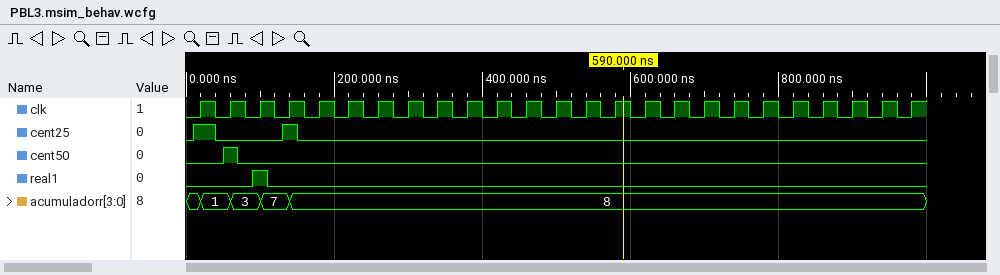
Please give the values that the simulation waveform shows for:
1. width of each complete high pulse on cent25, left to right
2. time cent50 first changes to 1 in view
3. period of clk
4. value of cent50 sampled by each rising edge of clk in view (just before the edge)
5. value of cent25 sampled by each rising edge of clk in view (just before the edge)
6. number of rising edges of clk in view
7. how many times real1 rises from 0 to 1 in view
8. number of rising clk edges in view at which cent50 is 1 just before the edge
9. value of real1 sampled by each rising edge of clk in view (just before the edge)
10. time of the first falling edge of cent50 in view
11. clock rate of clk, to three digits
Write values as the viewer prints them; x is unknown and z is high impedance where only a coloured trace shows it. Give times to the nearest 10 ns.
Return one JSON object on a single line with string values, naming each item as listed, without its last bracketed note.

{"width of each complete high pulse on cent25, left to right": "30 ns, 20 ns", "time cent50 first changes to 1 in view": "50 ns", "period of clk": "40 ns", "value of cent50 sampled by each rising edge of clk in view": "0 1 0 0 0 0 0 0 0 0 0 0 0 0 0 0 0 0 0 0 0 0 0 0 0", "value of cent25 sampled by each rising edge of clk in view": "1 0 0 1 0 0 0 0 0 0 0 0 0 0 0 0 0 0 0 0 0 0 0 0 0", "number of rising edges of clk in view": "25", "how many times real1 rises from 0 to 1 in view": "1", "number of rising clk edges in view at which cent50 is 1 just before the edge": "1", "value of real1 sampled by each rising edge of clk in view": "0 0 1 0 0 0 0 0 0 0 0 0 0 0 0 0 0 0 0 0 0 0 0 0 0", "time of the first falling edge of cent50 in view": "70 ns", "clock rate of clk, to three digits": "25.0 MHz"}
